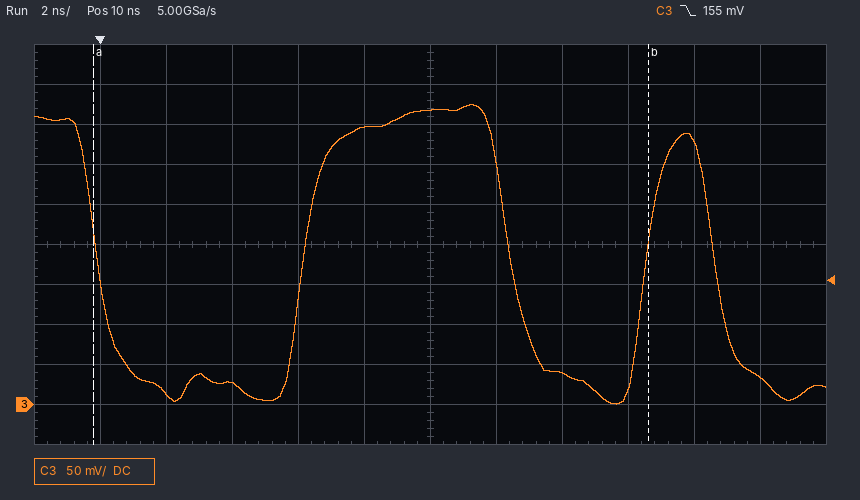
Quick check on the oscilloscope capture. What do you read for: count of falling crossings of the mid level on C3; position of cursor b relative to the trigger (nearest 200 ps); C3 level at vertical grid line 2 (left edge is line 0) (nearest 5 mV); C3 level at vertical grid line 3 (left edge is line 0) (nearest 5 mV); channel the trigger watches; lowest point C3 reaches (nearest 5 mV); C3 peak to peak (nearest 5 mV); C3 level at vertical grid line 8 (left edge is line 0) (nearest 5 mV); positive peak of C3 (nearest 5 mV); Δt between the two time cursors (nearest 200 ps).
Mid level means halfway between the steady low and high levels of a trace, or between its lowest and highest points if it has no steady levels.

3
+16.6 ns
15 mV
25 mV
C3
0 mV
375 mV
40 mV
375 mV
16.8 ns
